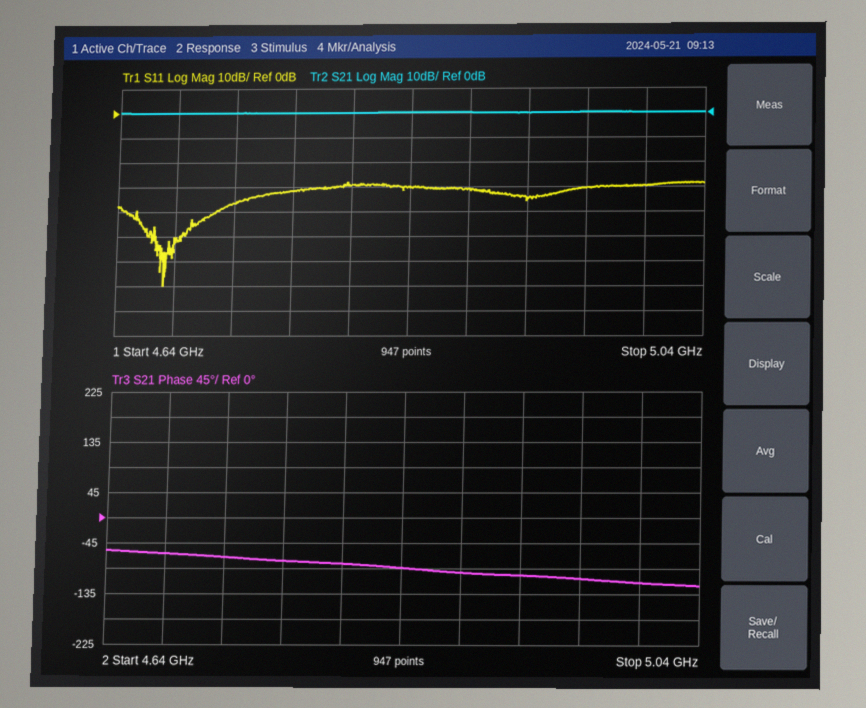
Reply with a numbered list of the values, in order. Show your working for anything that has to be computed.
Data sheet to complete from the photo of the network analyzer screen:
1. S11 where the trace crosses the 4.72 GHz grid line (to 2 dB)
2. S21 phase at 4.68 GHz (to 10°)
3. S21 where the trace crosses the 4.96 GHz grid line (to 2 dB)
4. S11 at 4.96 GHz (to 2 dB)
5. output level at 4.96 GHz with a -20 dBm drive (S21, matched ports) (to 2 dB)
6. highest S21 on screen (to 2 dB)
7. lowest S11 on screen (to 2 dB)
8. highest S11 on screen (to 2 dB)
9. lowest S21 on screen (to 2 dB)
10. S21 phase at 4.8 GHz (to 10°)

1. -36 dB
2. -60°
3. 0 dB
4. -30 dB
5. -20 dBm + (0 dB) = -20 dBm
6. 0 dB
7. -70 dB
8. -28 dB
9. 0 dB
10. -80°
